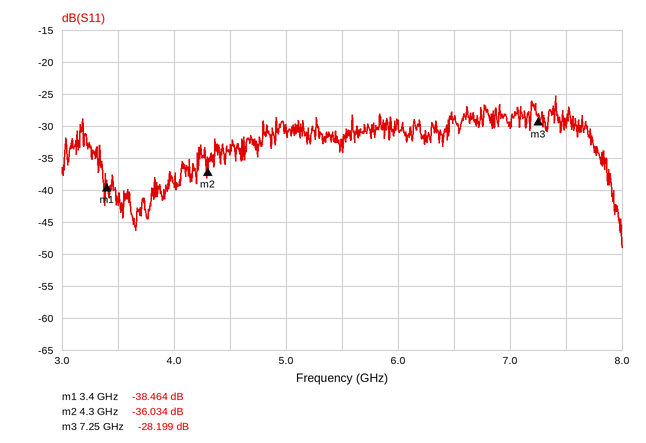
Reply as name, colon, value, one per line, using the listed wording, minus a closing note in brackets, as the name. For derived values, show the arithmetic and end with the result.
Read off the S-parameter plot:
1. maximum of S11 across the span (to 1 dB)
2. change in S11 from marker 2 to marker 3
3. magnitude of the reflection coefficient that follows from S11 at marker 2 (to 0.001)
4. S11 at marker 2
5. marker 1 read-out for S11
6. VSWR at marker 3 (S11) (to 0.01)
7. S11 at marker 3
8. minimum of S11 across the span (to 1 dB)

maximum of S11 across the span: -25 dB
change in S11 from marker 2 to marker 3: -28.199 − (-36.034) = 7.835 dB
magnitude of the reflection coefficient that follows from S11 at marker 2: 10^(-36.034/20) ≈ 0.016
S11 at marker 2: -36.034 dB
marker 1 read-out for S11: -38.464 dB
VSWR at marker 3 (S11): (1 + 0.0389)/(1 − 0.0389) ≈ 1.08
S11 at marker 3: -28.199 dB
minimum of S11 across the span: -49 dB
